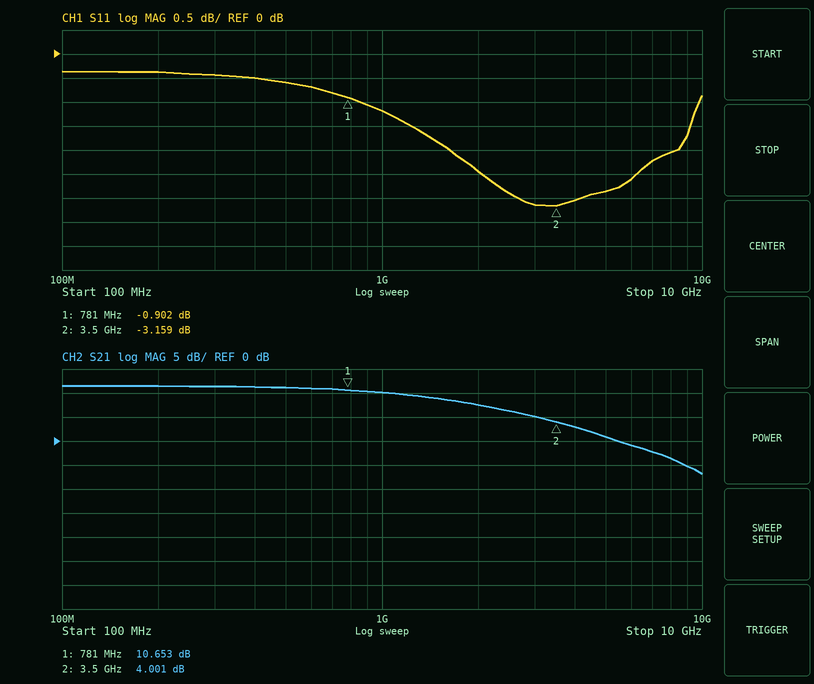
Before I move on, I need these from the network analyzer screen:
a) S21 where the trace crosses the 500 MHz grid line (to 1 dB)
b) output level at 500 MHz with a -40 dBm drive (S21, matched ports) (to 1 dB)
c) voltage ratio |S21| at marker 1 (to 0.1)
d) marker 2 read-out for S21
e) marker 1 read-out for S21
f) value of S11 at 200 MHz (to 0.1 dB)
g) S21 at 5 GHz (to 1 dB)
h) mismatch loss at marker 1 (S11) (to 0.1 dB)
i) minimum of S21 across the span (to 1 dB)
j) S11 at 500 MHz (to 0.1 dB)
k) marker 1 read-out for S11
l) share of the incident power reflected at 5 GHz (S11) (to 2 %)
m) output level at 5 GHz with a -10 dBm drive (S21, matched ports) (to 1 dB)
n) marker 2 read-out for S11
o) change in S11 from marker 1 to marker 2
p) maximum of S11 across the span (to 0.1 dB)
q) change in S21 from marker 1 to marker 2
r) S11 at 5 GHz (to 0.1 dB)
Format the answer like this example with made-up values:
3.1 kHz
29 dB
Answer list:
11 dB
-29 dBm
3.4
4.001 dB
10.653 dB
-0.4 dB
1 dB
7.3 dB
-7 dB
-0.6 dB
-0.902 dB
52 %
-9 dBm
-3.159 dB
-2.257 dB
-0.4 dB
-6.652 dB
-2.9 dB
